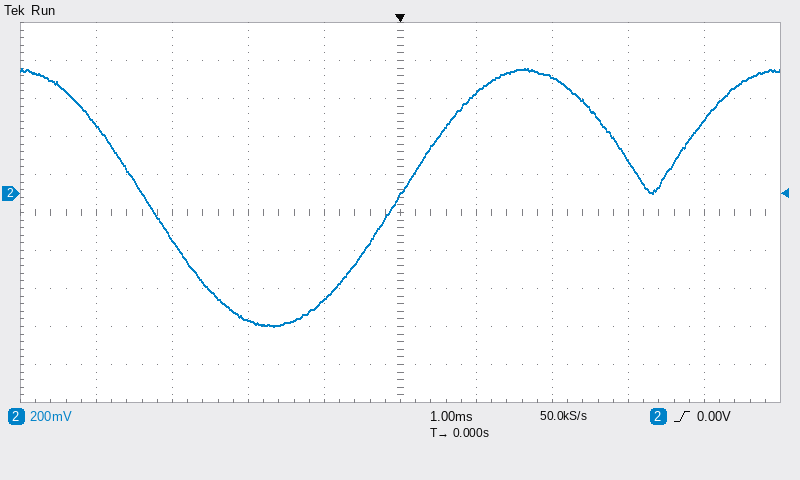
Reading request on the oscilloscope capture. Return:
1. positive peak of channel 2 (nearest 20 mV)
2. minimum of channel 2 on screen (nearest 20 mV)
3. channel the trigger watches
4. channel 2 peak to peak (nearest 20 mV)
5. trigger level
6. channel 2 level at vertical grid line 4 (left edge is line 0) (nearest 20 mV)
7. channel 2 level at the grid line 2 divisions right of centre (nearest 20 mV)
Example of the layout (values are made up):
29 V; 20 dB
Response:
660 mV; -700 mV; channel 2; 1.36 V; 0.00 V; -560 mV; 620 mV
